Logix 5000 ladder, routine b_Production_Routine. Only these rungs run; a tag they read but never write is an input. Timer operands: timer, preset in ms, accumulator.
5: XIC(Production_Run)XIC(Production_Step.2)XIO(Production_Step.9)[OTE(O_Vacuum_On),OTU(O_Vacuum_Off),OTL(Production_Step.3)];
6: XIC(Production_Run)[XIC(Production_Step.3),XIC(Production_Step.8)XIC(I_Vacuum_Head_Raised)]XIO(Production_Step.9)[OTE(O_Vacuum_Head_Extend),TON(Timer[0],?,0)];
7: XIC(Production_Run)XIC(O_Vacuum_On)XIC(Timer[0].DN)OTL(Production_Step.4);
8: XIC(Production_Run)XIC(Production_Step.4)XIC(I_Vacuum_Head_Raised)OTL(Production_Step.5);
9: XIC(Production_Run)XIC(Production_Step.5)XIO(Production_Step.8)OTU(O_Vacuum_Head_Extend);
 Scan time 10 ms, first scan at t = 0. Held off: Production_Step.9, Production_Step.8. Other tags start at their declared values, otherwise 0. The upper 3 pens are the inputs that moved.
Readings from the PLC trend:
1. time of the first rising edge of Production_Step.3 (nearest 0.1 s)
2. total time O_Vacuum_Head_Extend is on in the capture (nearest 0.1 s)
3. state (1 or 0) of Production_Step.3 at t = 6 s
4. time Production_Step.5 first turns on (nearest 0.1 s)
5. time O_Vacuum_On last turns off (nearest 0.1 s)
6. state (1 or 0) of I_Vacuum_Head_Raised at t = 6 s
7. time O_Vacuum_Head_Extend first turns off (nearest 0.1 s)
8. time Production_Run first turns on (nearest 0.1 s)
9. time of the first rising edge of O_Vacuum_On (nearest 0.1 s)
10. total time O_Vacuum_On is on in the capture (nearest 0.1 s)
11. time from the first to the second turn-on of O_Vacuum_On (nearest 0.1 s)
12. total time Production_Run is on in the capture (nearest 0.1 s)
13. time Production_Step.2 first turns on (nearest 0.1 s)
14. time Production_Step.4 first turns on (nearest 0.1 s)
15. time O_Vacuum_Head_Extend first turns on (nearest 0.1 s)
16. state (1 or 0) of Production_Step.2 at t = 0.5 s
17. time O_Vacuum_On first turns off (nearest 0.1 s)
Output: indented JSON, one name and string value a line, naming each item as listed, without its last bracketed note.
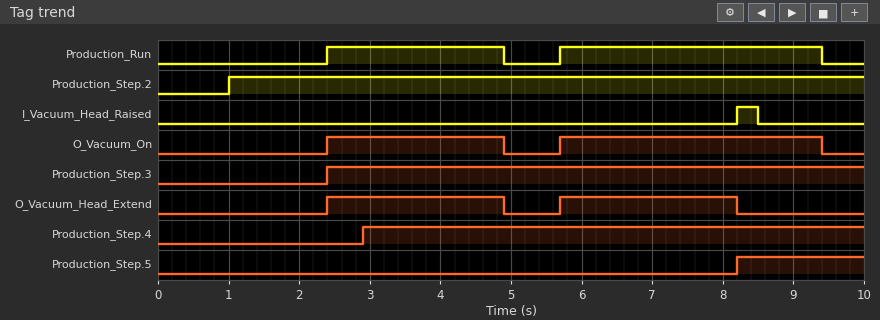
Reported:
{
  "time of the first rising edge of Production_Step.3": "2.4 s",
  "total time O_Vacuum_Head_Extend is on in the capture": "5.0 s",
  "state (1 or 0) of Production_Step.3 at t = 6 s": "1",
  "time Production_Step.5 first turns on": "8.2 s",
  "time O_Vacuum_On last turns off": "9.4 s",
  "state (1 or 0) of I_Vacuum_Head_Raised at t = 6 s": "0",
  "time O_Vacuum_Head_Extend first turns off": "4.9 s",
  "time Production_Run first turns on": "2.4 s",
  "time of the first rising edge of O_Vacuum_On": "2.4 s",
  "total time O_Vacuum_On is on in the capture": "6.2 s",
  "time from the first to the second turn-on of O_Vacuum_On": "3.3 s",
  "total time Production_Run is on in the capture": "6.2 s",
  "time Production_Step.2 first turns on": "1.0 s",
  "time Production_Step.4 first turns on": "2.9 s",
  "time O_Vacuum_Head_Extend first turns on": "2.4 s",
  "state (1 or 0) of Production_Step.2 at t = 0.5 s": "0",
  "time O_Vacuum_On first turns off": "4.9 s"
}
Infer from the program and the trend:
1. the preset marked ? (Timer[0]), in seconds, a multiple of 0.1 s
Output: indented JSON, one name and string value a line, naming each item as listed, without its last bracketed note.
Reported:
{
  "the preset marked ? (Timer[0]), in seconds, a multiple of 0.1 s": "0.5 s"
}
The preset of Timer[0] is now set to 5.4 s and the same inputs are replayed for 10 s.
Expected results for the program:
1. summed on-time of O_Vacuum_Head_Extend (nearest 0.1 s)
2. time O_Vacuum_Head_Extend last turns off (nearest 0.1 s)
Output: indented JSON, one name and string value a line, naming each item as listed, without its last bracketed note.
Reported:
{
  "summed on-time of O_Vacuum_Head_Extend": "6.2 s",
  "time O_Vacuum_Head_Extend last turns off": "9.4 s"
}
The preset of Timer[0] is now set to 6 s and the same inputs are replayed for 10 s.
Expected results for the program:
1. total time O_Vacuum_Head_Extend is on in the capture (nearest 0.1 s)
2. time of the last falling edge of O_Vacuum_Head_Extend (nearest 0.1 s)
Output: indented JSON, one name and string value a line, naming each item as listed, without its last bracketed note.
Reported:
{
  "total time O_Vacuum_Head_Extend is on in the capture": "6.2 s",
  "time of the last falling edge of O_Vacuum_Head_Extend": "9.4 s"
}
